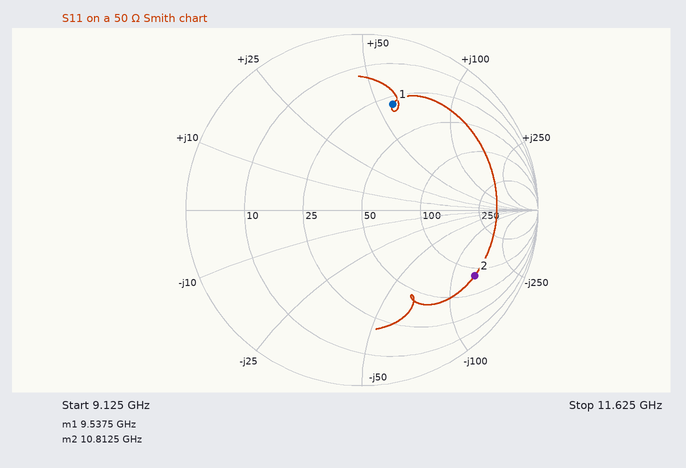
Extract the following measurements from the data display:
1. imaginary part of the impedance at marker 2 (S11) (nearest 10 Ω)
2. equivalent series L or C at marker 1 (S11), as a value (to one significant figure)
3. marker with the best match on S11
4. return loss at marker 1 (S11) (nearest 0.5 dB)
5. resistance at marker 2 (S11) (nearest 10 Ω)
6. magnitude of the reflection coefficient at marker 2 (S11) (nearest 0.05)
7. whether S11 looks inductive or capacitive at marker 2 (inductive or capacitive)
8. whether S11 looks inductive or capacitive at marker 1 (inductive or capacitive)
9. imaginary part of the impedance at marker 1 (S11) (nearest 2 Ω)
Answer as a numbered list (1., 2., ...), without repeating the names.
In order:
1. -140 Ω
2. 1.0 nH
3. marker 1
4. 4.0 dB
5. 80 Ω
6. 0.75
7. capacitive
8. inductive
9. +58 Ω
